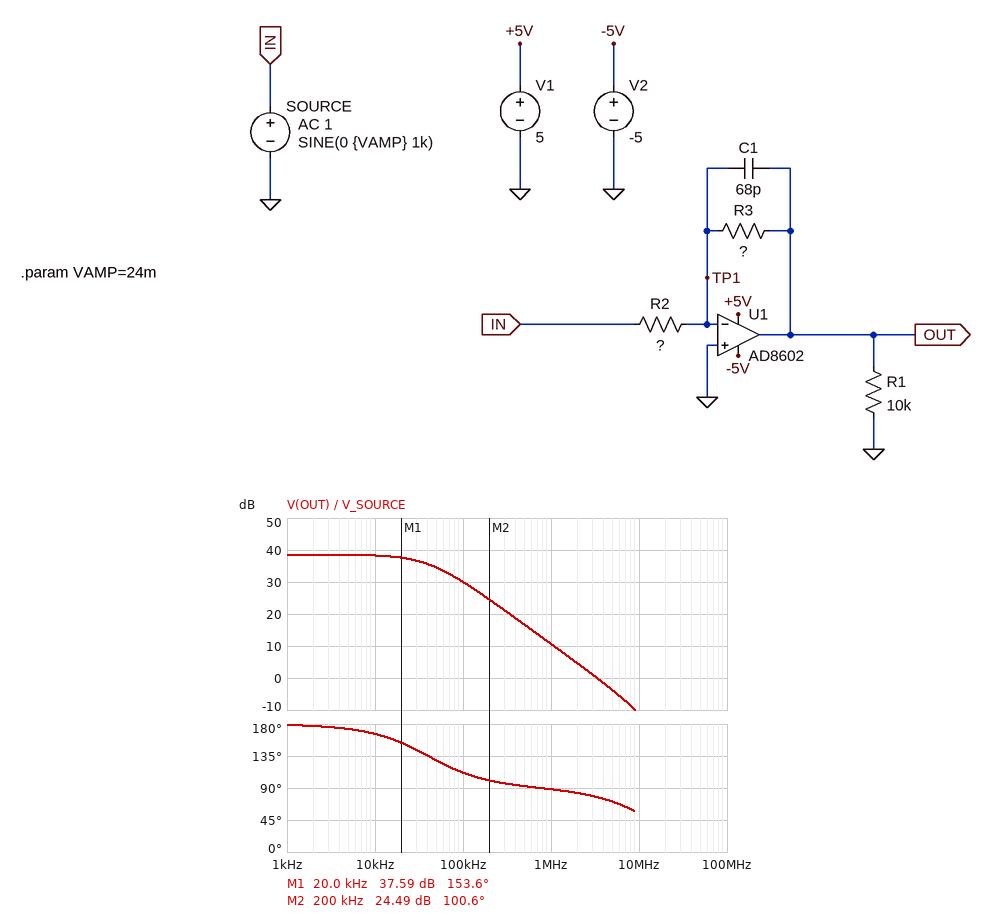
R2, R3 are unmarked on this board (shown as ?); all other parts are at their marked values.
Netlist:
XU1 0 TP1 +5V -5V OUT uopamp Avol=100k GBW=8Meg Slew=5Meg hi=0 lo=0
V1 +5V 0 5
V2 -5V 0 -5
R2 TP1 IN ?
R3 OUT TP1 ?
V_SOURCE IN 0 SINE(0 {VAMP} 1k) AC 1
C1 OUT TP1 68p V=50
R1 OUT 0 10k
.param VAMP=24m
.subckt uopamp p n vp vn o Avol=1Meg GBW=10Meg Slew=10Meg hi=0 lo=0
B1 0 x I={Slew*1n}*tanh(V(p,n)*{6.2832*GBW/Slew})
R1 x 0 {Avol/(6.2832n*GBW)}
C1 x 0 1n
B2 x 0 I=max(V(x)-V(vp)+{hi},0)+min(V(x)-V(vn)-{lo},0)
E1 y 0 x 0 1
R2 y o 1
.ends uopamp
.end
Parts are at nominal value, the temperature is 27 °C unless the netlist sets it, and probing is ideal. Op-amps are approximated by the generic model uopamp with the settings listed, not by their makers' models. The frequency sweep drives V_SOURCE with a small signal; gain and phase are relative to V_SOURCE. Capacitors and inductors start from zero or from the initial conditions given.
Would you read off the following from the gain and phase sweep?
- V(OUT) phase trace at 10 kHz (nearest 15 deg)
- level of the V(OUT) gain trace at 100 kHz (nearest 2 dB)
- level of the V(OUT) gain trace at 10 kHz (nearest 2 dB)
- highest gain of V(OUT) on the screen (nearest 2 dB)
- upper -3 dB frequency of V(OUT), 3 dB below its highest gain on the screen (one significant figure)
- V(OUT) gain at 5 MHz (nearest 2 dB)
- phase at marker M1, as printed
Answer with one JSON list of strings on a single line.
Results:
["165 deg", "30 dB", "38 dB", "38 dB", "40 kHz", "-4 dB", "153.6 deg"]
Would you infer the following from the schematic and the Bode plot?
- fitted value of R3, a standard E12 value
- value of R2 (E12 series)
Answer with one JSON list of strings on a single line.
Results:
["33 kΩ", "390 Ω"]
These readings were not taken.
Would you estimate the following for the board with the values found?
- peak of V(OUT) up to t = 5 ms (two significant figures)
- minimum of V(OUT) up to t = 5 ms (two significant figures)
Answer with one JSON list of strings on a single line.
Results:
["2.0 V", "-2.0 V"]
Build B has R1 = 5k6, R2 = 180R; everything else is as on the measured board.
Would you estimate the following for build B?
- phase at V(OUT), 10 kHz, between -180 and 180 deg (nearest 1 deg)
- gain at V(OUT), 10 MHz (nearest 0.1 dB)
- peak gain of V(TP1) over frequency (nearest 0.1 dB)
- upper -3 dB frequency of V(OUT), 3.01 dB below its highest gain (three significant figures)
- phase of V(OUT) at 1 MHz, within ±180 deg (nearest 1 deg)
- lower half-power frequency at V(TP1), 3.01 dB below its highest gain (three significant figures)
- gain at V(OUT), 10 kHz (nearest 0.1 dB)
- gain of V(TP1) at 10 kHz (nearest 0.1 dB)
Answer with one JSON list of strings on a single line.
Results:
["160 deg", "-7.0 dB", "-4.2 dB", "27.0 kHz", "89 deg", "26.9 kHz", "44.7 dB", "-13.4 dB"]
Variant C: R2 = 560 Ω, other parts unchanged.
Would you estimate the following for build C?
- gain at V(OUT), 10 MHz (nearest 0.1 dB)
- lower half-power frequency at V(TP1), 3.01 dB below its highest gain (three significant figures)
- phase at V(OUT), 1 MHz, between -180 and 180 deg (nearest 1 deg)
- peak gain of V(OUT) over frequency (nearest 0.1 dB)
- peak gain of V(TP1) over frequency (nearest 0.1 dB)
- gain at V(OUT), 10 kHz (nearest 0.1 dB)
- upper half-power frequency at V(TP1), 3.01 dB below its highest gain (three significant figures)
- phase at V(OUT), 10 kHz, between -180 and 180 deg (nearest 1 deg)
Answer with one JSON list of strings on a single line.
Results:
["-13.4 dB", "46.2 kHz", "88 deg", "35.4 dB", "-9.3 dB", "35.2 dB", "12.3 MHz", "168 deg"]
